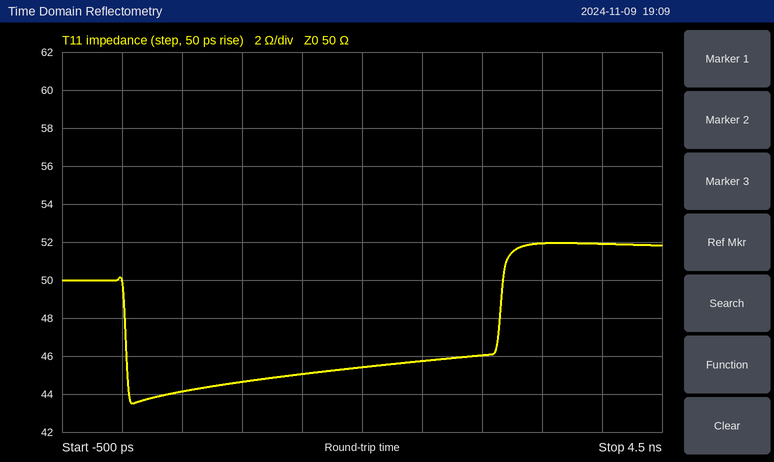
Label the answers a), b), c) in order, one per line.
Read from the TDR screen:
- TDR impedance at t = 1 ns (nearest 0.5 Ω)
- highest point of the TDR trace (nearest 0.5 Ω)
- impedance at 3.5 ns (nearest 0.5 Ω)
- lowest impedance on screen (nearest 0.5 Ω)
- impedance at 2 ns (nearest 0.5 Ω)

a) 44.5 Ω
b) 52.0 Ω
c) 52.0 Ω
d) 43.5 Ω
e) 45.5 Ω
